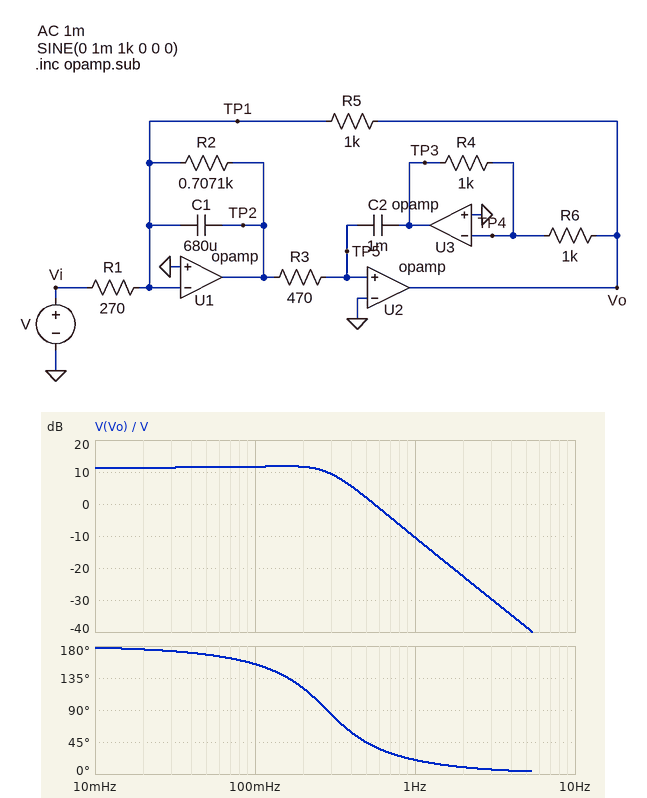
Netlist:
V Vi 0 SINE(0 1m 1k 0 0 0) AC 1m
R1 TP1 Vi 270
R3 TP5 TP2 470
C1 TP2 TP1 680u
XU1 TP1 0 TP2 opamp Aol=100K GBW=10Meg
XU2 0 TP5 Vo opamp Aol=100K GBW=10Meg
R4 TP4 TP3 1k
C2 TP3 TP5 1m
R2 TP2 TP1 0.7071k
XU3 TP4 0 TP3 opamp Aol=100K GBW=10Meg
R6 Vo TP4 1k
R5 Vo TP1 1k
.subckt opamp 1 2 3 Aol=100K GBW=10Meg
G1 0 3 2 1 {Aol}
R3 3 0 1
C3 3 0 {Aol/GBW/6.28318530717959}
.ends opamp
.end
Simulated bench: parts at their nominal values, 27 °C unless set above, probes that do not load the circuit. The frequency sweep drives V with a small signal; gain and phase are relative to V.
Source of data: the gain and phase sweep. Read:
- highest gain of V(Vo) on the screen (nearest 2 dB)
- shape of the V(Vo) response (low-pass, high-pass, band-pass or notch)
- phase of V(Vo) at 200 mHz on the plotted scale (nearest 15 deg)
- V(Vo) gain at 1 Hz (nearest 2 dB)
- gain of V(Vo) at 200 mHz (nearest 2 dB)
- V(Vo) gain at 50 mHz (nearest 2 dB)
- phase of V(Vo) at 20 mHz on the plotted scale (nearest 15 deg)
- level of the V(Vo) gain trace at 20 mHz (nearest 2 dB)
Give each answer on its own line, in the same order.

12 dB
low-pass
120 deg
-10 dB
12 dB
12 dB
180 deg
12 dB
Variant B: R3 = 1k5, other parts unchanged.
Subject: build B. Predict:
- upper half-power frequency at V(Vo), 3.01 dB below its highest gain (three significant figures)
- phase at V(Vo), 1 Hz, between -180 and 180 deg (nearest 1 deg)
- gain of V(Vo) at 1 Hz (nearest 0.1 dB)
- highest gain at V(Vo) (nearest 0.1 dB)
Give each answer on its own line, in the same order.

94.6 mHz
19 deg
-21.0 dB
11.4 dB
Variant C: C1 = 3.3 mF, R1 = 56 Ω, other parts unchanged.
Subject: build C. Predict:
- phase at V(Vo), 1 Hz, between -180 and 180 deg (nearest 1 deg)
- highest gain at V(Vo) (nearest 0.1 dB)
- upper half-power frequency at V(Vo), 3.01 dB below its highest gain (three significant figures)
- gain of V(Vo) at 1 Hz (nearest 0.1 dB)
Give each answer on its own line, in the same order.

4 deg
30.8 dB
150 mHz
-10.6 dB
